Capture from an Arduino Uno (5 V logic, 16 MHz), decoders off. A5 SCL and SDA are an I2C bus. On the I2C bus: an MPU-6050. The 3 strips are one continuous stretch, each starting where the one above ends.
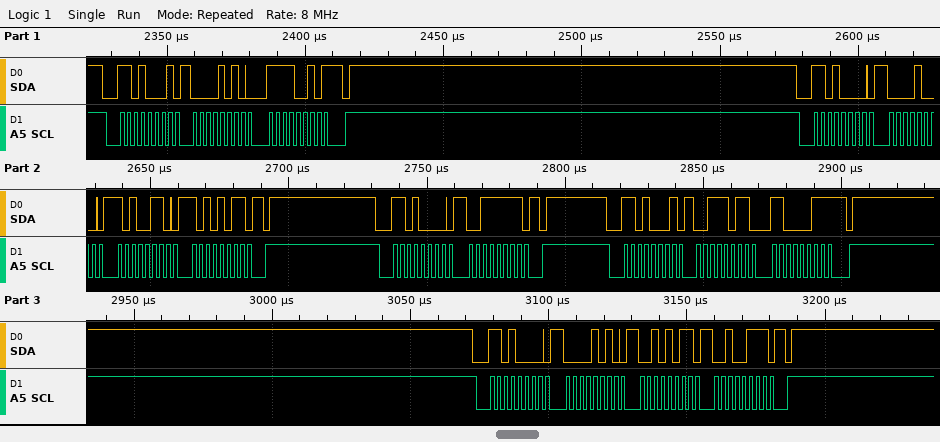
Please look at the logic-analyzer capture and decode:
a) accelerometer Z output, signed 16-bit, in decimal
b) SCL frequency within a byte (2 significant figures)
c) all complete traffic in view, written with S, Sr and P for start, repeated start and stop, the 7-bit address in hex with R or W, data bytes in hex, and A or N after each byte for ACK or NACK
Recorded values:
15299
400 kHz
S 68R A 0A A F2 N P S 68W A 08 A A6 A AB A P S 68W A 3F A P S 68R A 3B A C3 N P S 68W A 0A A 2B A 27 A P
